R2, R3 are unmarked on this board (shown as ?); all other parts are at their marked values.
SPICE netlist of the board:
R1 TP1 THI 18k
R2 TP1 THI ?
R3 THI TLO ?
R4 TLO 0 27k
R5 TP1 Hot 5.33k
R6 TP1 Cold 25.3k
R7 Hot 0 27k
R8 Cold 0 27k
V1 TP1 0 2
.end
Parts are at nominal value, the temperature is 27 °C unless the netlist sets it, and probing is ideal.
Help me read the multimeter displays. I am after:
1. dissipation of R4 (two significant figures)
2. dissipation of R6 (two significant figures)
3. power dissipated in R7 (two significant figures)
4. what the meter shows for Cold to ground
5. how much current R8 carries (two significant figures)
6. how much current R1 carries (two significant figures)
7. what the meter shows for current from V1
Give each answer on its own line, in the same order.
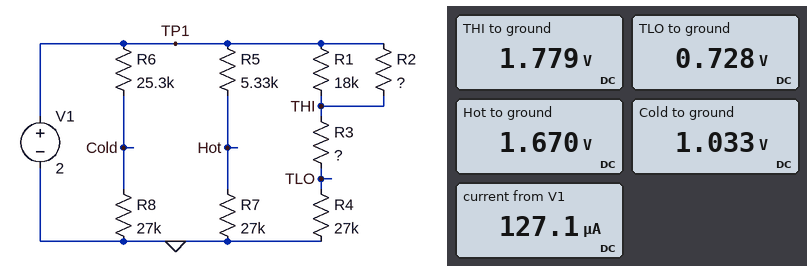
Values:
20 µW
37 µW
100 µW
1.033 V
38 µA
12 µA
127.1 µA
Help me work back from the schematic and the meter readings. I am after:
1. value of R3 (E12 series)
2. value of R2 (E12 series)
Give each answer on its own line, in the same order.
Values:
39 kΩ
15 kΩ
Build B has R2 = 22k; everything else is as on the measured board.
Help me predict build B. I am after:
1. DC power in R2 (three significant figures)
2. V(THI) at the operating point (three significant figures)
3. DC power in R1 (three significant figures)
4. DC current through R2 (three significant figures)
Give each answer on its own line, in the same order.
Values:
3.09 µW
1.74 V
3.78 µW
11.9 µA
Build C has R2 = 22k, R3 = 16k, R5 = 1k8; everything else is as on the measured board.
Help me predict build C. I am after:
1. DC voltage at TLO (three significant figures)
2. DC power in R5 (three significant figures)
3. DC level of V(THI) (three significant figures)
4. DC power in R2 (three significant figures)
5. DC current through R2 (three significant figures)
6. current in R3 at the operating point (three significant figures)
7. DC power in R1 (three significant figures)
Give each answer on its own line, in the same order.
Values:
1.02 V
8.68 µW
1.63 V
6.37 µW
17.0 µA
37.8 µA
7.78 µW
